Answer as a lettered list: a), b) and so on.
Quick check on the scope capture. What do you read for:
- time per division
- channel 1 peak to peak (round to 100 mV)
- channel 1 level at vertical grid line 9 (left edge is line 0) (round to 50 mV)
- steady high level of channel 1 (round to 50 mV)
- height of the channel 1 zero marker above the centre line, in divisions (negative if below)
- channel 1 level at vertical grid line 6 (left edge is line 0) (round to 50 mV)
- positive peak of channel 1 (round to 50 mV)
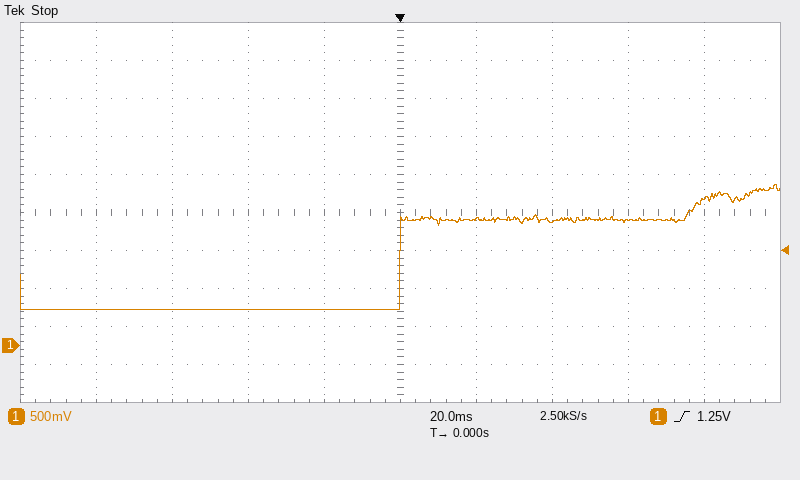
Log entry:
a) 20 ms
b) 1.60 V
c) 1.90 V
d) 1.65 V
e) -3.5 div
f) 1.65 V
g) 2.10 V
